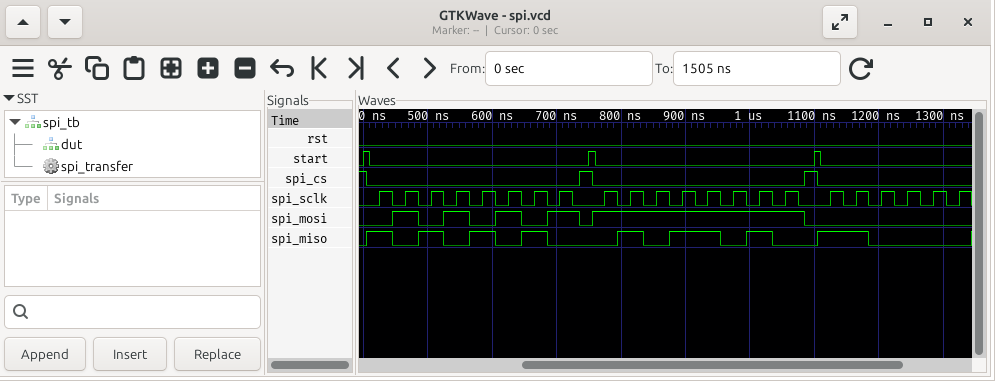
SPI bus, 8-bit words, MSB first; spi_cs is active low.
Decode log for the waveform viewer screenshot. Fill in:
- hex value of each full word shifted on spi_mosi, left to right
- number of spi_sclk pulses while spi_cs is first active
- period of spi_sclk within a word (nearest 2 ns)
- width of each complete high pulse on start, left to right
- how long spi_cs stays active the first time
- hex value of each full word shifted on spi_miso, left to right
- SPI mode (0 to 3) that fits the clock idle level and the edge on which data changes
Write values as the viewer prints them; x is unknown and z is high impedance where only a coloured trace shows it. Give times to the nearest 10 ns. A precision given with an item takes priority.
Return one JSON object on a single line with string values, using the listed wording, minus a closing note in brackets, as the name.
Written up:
{"hex value of each full word shifted on spi_mosi, left to right": "55, FF", "number of spi_sclk pulses while spi_cs is first active": "8", "period of spi_sclk within a word": "40 ns", "width of each complete high pulse on start, left to right": "10 ns, 10 ns, 10 ns", "how long spi_cs stays active the first time": "330 ns", "hex value of each full word shifted on spi_miso, left to right": "AA, 5A", "SPI mode (0 to 3) that fits the clock idle level and the edge on which data changes": "0"}
